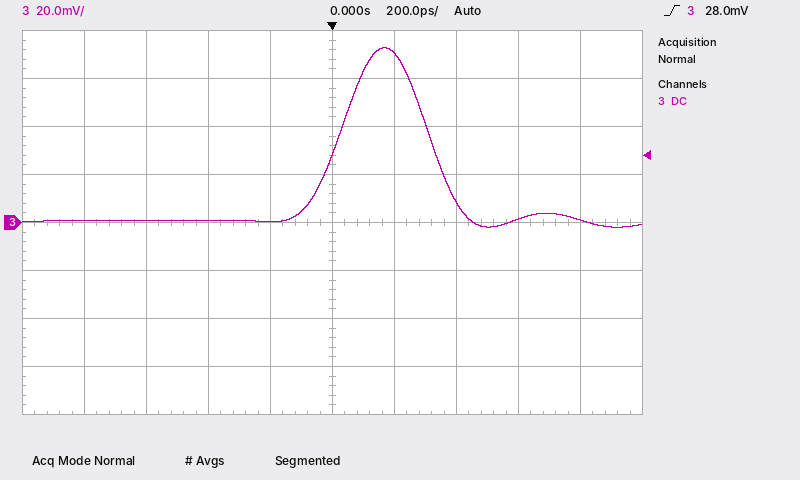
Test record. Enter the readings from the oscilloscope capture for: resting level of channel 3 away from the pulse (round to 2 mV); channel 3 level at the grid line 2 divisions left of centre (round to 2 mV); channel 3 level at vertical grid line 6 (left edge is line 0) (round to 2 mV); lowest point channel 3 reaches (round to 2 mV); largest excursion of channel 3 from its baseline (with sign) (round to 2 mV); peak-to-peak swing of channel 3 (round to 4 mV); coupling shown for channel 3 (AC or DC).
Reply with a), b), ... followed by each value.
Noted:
a) 0 mV
b) 0 mV
c) 70 mV
d) -2 mV
e) +72 mV
f) 76 mV
g) DC
